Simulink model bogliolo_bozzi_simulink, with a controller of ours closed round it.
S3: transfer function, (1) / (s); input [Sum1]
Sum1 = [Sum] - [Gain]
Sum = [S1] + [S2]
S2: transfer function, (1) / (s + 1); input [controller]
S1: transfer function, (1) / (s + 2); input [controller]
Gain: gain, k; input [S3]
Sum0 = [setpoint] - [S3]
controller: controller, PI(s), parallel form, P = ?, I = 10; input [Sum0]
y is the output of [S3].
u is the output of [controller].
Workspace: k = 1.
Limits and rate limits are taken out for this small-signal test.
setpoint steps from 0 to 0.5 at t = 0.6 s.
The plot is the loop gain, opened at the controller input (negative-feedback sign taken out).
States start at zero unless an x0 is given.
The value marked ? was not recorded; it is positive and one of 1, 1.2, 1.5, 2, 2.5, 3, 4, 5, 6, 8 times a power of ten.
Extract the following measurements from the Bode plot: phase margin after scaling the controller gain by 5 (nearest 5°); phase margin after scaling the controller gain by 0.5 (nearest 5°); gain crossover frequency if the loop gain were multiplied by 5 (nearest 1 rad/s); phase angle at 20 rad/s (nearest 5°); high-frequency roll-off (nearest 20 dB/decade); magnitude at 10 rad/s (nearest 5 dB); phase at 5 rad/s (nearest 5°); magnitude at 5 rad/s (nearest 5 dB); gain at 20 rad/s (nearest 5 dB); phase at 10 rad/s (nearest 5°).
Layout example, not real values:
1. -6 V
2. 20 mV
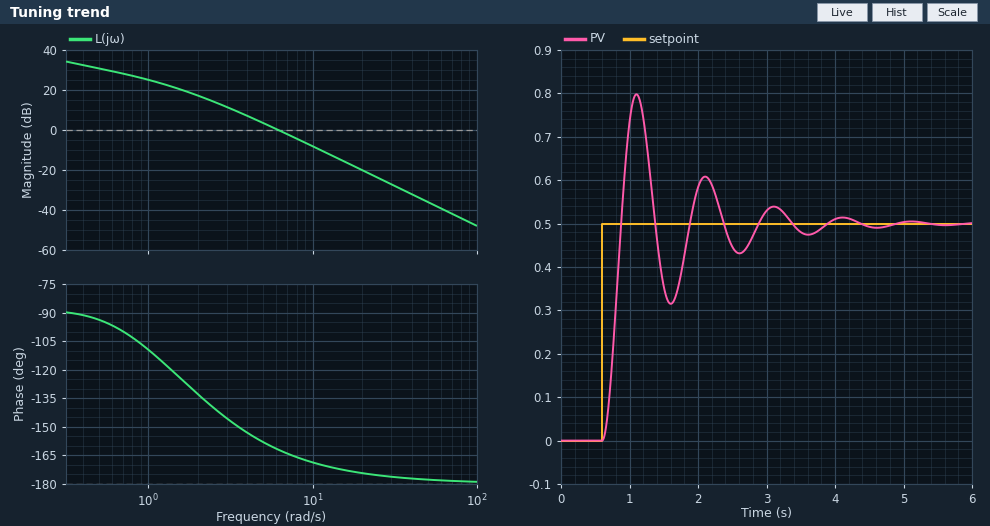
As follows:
1. 10°
2. 25°
3. 14 rad/s
4. -175°
5. -40 dB/decade
6. -10 dB
7. -160°
8. 5 dB
9. -20 dB
10. -170°
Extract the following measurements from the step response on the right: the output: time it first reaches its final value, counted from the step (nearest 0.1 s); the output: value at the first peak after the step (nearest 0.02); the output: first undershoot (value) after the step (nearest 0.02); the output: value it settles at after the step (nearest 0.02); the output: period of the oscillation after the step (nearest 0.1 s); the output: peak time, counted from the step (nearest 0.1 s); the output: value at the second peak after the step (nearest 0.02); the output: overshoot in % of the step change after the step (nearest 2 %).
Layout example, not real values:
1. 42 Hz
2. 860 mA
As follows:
1. 0.3 s
2. 0.80
3. 0.32
4. 0.50
5. 1.0 s
6. 0.5 s
7. 0.60
8. 60 %
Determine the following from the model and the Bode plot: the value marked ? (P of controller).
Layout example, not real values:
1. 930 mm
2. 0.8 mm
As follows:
1. 20
